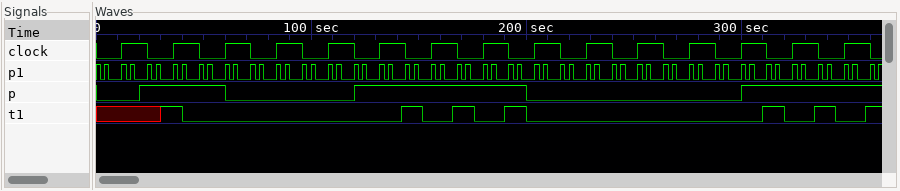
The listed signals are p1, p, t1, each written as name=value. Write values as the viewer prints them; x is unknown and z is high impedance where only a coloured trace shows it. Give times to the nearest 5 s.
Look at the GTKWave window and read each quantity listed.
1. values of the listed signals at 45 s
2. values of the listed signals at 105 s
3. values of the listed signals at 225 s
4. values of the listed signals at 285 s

p1=0, p=1, t1=0
p1=0, p=0, t1=0
p1=0, p=0, t1=0
p1=0, p=0, t1=0
